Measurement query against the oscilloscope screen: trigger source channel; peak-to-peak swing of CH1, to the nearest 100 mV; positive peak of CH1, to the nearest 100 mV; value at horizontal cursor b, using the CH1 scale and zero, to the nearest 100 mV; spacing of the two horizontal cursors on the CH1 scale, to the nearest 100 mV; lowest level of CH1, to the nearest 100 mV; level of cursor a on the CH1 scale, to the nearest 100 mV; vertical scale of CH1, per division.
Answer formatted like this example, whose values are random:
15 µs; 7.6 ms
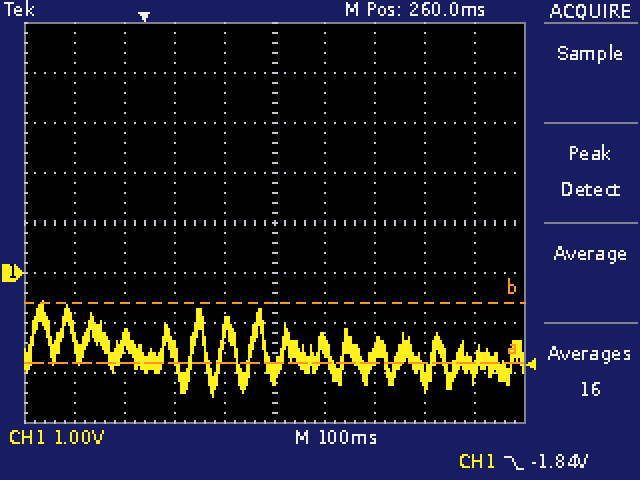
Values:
CH1; 1.9 V; -600 mV; -600 mV; 1.2 V; -2.5 V; -1.8 V; 1 V
